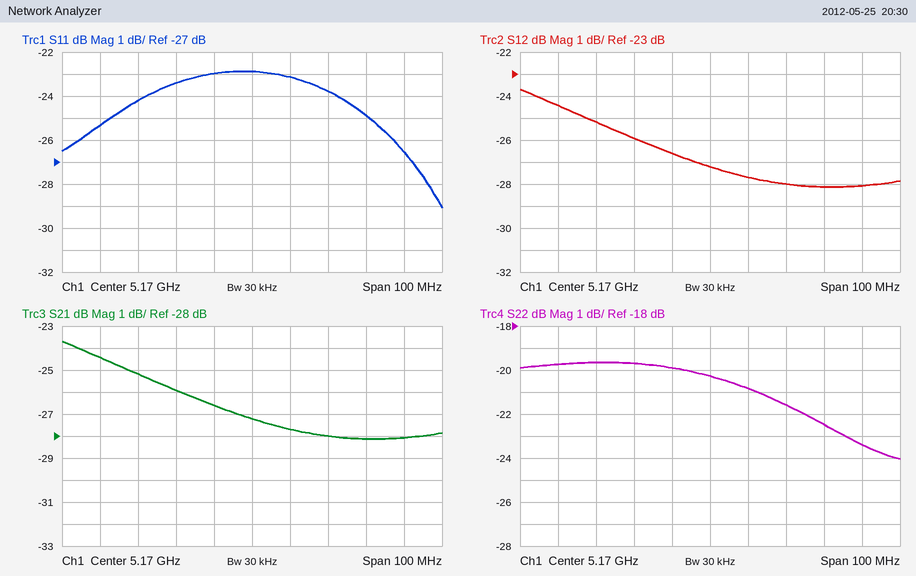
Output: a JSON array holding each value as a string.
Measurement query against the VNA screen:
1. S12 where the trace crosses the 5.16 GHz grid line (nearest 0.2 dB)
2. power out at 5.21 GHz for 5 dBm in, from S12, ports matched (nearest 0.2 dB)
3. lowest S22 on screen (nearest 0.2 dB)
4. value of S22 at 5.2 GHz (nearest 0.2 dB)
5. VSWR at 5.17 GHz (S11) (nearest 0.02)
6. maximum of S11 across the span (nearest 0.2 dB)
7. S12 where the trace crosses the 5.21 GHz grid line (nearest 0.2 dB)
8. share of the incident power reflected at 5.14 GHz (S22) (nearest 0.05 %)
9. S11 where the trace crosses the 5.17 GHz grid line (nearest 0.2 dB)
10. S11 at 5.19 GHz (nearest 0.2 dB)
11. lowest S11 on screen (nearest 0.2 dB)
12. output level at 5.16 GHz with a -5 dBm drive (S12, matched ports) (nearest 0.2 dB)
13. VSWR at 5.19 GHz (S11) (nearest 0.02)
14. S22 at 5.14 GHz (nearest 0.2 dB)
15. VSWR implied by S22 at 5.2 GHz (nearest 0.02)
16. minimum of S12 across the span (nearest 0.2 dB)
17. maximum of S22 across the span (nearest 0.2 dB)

["-26.6 dB", "-23.0 dBm", "-24.0 dB", "-22.4 dB", "1.16", "-22.8 dB", "-28.0 dB", "1.10 %", "-22.8 dB", "-23.8 dB", "-29.0 dB", "-31.6 dBm", "1.14", "-19.6 dB", "1.16", "-28.2 dB", "-19.6 dB"]
